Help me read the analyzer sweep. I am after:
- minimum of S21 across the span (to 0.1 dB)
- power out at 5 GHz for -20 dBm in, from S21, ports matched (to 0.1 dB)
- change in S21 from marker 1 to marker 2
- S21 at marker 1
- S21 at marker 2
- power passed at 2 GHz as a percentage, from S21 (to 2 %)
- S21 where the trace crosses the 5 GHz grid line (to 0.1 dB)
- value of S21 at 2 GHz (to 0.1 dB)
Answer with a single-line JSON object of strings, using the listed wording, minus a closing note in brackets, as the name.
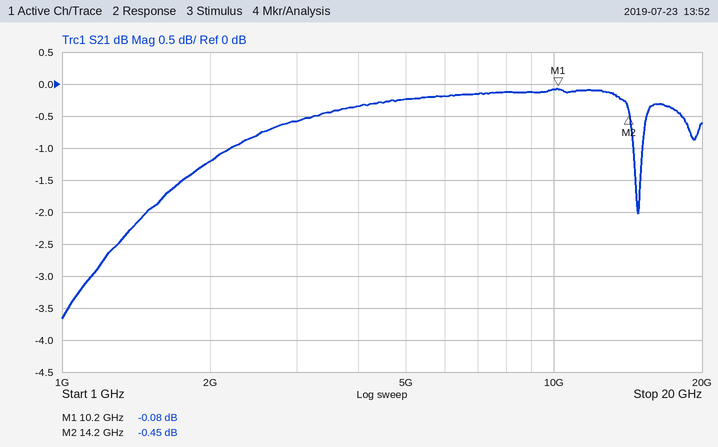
{"minimum of S21 across the span": "-3.7 dB", "power out at 5 GHz for -20 dBm in, from S21, ports matched": "-20.2 dBm", "change in S21 from marker 1 to marker 2": "-0.37 dB", "S21 at marker 1": "-0.08 dB", "S21 at marker 2": "-0.45 dB", "power passed at 2 GHz as a percentage, from S21": "76 %", "S21 where the trace crosses the 5 GHz grid line": "-0.2 dB", "value of S21 at 2 GHz": "-1.2 dB"}
